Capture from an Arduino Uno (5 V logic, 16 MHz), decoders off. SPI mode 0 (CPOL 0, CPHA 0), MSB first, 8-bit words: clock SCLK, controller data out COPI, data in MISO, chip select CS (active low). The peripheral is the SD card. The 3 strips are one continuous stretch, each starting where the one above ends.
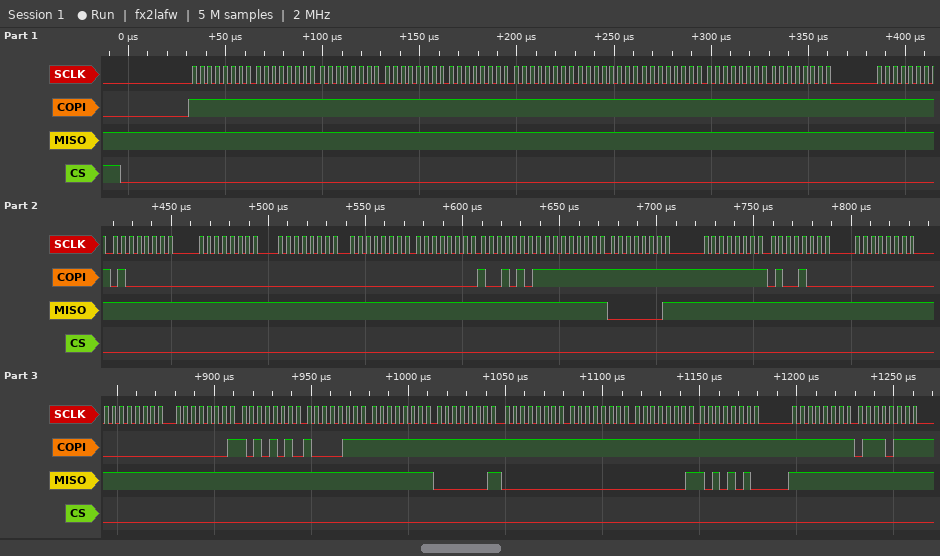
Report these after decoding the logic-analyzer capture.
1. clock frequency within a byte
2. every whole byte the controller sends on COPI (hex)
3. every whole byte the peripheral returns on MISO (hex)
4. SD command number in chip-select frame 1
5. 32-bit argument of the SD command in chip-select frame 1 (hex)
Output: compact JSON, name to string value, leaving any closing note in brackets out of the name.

{"clock frequency within a byte": "250 kHz", "every whole byte the controller sends on COPI": "FF FF FF FF FF FF FF FF FF FF FF 40 00 00 00 00 95 FF FF FF 48 00 00 01 AA 87 FF FF FF FF FF FF FF 77", "every whole byte the peripheral returns on MISO": "FF FF FF FF FF FF FF FF FF FF FF FF FF FF FF FF FF FF 01 FF FF FF FF FF FF FF FF 01 00 00 01 AA FF FF", "SD command number in chip-select frame 1": "CMD0", "32-bit argument of the SD command in chip-select frame 1": "0x00000000"}
